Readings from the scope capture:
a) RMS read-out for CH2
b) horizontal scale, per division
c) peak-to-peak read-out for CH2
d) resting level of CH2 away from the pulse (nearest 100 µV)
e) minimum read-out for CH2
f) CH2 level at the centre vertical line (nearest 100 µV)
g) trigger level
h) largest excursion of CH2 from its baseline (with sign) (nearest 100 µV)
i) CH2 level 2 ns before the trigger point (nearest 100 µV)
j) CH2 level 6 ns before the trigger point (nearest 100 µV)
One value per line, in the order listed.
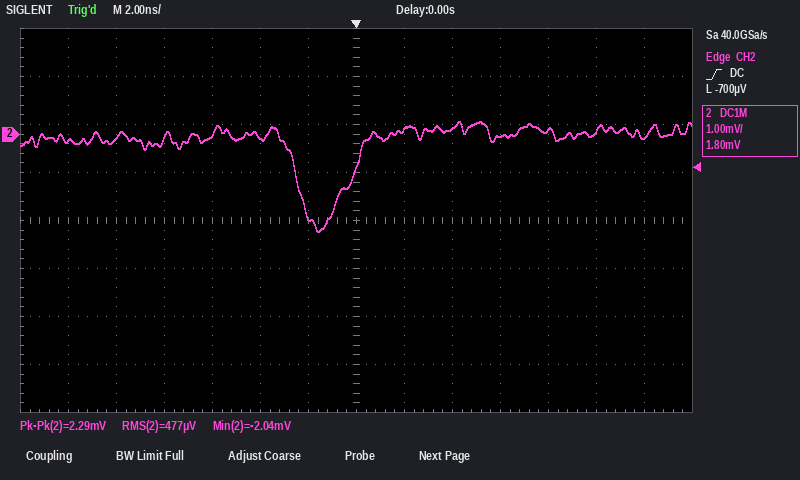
477 µV
2 ns
2.29 mV
0.0 mV
-2.04 mV
-700 µV
-700 µV
-2.0 mV
-1.7 mV
0.0 mV
